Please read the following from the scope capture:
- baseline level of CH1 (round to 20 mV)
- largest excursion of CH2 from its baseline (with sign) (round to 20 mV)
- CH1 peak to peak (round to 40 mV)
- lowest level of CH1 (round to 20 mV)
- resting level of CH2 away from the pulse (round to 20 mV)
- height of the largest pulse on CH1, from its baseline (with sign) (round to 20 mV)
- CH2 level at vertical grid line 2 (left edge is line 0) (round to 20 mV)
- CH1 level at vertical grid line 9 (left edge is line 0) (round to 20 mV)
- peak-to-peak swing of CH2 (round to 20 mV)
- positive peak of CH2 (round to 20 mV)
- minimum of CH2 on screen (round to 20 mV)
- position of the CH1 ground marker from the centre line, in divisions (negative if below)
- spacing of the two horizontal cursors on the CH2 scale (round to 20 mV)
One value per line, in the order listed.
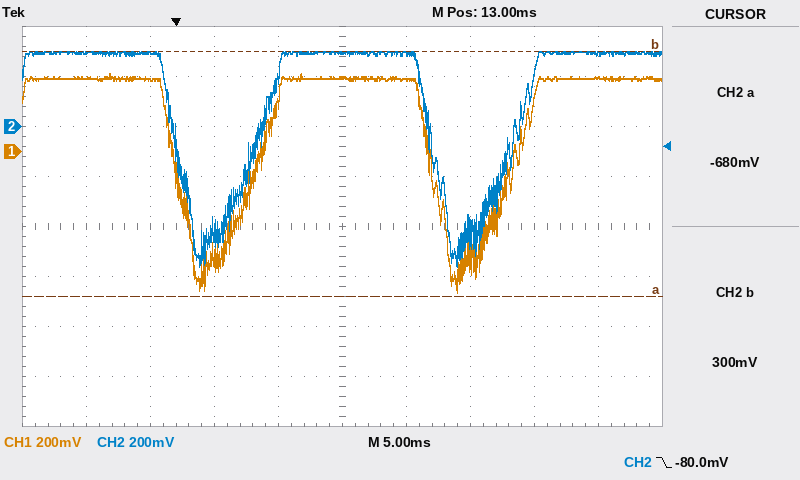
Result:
300 mV
-860 mV
880 mV
-560 mV
300 mV
-860 mV
300 mV
300 mV
860 mV
300 mV
-560 mV
+1.5 div
980 mV
